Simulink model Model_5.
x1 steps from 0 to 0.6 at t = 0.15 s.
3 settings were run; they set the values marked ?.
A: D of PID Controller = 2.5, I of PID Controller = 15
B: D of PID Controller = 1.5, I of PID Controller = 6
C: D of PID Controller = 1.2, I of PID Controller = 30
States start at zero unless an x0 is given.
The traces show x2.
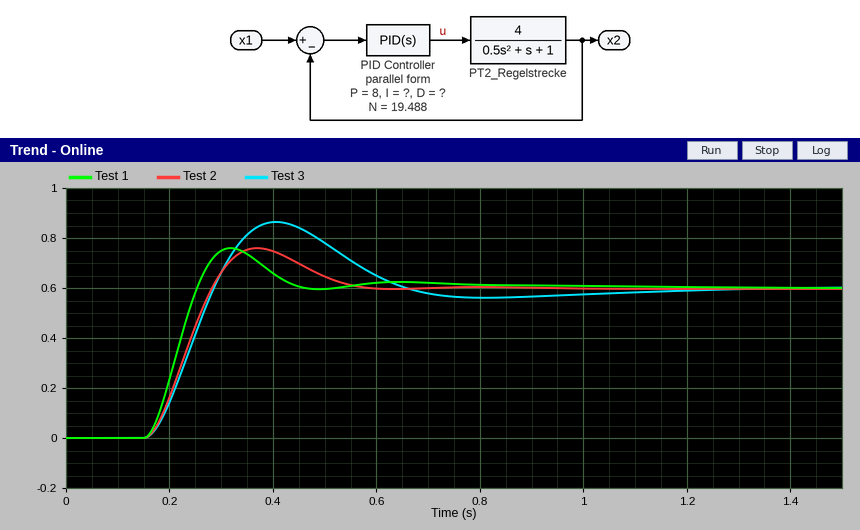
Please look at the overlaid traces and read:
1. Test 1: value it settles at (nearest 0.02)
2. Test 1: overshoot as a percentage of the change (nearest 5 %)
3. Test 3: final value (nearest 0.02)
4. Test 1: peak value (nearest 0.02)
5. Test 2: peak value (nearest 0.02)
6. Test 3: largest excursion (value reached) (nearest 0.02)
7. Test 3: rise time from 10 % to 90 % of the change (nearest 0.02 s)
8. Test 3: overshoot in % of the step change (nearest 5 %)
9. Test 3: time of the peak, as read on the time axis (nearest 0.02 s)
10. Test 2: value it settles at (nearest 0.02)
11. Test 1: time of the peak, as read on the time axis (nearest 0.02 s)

0.60
25 %
0.60
0.76
0.76
0.86
0.10 s
45 %
0.40 s
0.60
0.32 s
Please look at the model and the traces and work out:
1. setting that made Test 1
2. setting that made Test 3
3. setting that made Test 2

A
C
B
